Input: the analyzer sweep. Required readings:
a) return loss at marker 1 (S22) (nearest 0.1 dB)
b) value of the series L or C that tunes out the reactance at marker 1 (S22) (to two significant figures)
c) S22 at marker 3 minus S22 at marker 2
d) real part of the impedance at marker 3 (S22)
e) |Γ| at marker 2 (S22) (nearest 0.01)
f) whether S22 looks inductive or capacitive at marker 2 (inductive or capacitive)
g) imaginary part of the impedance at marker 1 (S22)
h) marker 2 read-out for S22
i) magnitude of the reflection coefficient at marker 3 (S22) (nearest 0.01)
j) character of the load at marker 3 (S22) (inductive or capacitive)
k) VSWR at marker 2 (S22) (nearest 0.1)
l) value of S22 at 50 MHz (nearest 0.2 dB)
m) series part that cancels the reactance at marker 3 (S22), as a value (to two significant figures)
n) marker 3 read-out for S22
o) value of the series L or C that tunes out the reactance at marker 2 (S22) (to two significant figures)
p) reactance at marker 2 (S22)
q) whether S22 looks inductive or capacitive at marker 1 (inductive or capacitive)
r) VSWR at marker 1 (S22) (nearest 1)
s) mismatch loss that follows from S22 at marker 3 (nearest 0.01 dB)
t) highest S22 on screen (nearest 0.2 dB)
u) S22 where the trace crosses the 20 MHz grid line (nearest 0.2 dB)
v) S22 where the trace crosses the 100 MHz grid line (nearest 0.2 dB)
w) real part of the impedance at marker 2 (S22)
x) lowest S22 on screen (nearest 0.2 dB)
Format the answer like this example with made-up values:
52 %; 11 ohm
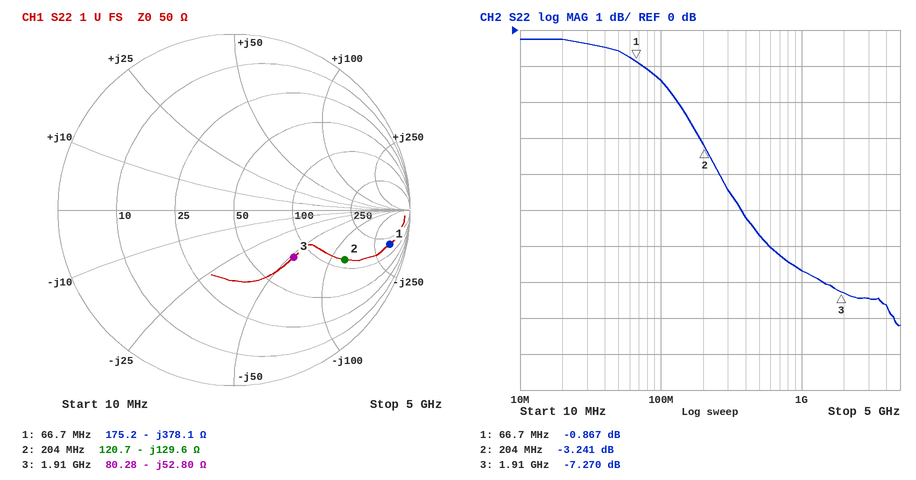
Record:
0.9 dB; 900 nH; -4.029 dB; 80.28 Ω; 0.69; capacitive; -378.1 Ω; -3.241 dB; 0.43; capacitive; 5.4; -0.6 dB; 4.4 nH; -7.270 dB; 100 nH; -129.6 Ω; capacitive; 20; 0.90 dB; -0.2 dB; -0.2 dB; -1.4 dB; 120.7 Ω; -8.2 dB
